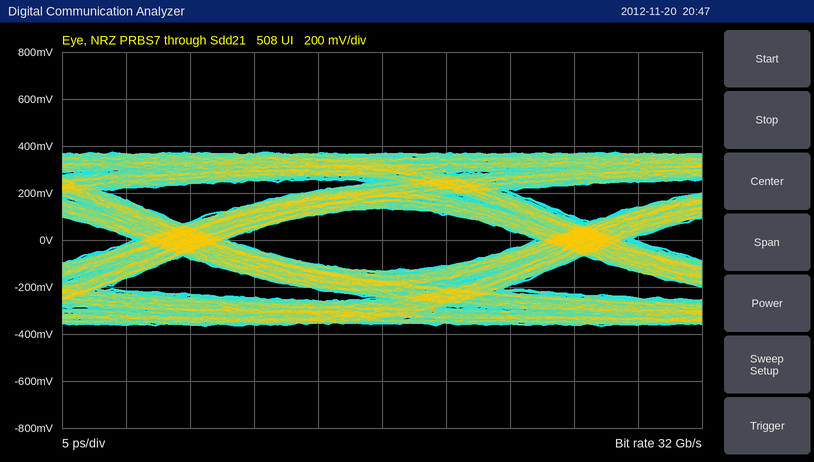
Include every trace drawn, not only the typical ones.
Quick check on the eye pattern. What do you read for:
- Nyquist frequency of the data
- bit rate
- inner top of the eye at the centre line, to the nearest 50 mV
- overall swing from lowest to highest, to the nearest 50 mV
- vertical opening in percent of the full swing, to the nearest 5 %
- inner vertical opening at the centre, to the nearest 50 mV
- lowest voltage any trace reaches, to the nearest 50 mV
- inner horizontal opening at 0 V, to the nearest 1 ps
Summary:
16 GHz
32 Gb/s
150 mV
750 mV
35 %
250 mV
-350 mV
24 ps
